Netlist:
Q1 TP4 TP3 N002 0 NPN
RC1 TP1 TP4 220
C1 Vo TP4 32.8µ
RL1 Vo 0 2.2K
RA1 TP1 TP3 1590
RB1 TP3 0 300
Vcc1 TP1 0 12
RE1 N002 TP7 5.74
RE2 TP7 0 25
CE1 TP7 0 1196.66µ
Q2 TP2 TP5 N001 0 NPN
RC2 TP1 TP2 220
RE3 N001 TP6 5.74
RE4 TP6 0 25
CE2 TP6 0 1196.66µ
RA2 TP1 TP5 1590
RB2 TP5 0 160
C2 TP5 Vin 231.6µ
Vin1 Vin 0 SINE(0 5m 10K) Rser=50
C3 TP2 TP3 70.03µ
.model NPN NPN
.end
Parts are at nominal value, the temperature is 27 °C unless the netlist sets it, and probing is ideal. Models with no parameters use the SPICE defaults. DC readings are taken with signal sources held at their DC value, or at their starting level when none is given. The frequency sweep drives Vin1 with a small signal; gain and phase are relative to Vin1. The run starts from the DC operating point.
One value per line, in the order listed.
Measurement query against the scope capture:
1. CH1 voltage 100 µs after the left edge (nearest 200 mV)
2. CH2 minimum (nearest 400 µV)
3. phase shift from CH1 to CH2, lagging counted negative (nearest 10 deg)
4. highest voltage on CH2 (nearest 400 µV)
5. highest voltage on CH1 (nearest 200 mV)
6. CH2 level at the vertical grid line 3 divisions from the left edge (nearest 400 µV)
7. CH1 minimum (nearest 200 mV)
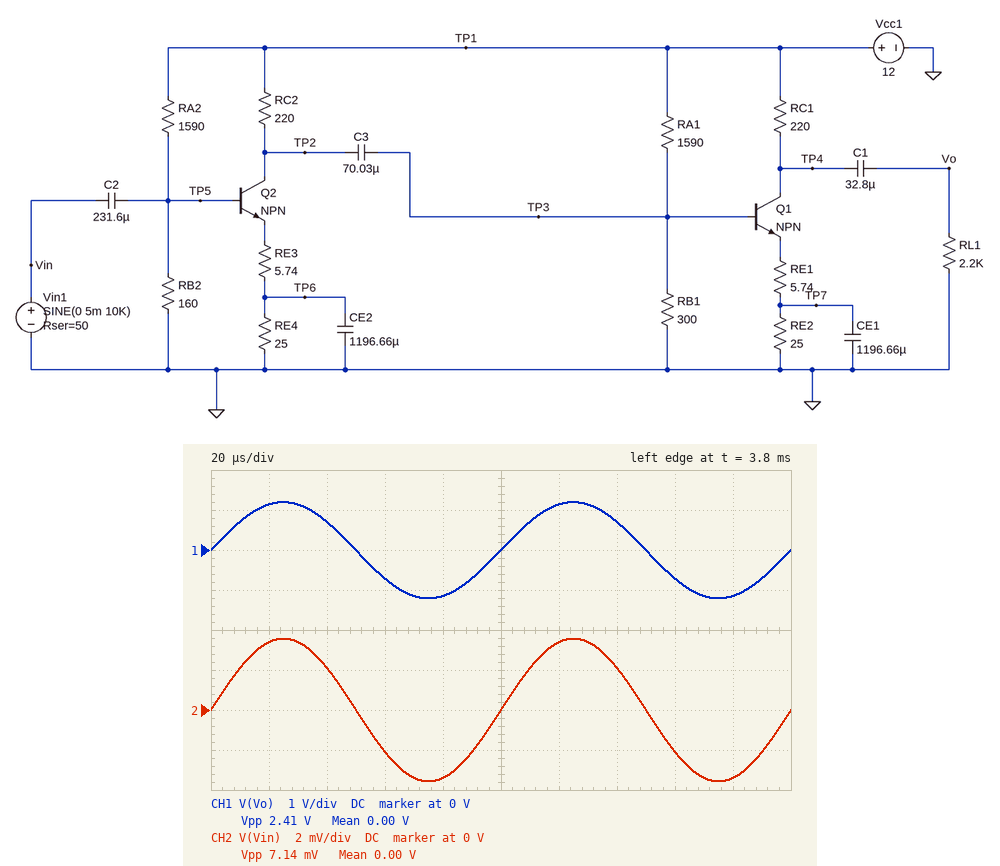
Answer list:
0 V
-3.6 mV
0 deg
3.6 mV
1.2 V
-2.0 mV
-1.2 V
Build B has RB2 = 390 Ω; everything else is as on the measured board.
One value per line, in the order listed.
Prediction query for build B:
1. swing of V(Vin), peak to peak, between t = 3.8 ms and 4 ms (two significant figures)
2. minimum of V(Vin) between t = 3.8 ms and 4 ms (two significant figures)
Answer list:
8.1 mV
-4.0 mV
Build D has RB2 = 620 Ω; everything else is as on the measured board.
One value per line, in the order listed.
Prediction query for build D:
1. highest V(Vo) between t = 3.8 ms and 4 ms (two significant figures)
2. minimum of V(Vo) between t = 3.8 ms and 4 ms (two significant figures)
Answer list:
20 mV
-21 mV
